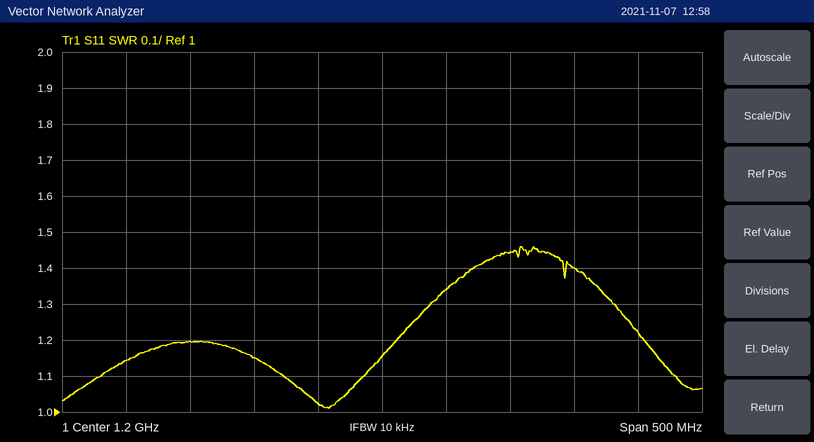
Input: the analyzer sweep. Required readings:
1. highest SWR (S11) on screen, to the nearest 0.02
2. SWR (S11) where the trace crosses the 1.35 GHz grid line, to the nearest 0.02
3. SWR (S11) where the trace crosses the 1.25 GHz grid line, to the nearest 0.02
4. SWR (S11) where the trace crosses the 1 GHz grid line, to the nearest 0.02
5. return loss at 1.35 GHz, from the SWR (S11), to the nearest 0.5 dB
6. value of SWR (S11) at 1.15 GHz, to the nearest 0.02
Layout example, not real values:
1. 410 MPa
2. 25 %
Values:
1. 1.46
2. 1.40
3. 1.34
4. 1.14
5. 15.5 dB
6. 1.02
